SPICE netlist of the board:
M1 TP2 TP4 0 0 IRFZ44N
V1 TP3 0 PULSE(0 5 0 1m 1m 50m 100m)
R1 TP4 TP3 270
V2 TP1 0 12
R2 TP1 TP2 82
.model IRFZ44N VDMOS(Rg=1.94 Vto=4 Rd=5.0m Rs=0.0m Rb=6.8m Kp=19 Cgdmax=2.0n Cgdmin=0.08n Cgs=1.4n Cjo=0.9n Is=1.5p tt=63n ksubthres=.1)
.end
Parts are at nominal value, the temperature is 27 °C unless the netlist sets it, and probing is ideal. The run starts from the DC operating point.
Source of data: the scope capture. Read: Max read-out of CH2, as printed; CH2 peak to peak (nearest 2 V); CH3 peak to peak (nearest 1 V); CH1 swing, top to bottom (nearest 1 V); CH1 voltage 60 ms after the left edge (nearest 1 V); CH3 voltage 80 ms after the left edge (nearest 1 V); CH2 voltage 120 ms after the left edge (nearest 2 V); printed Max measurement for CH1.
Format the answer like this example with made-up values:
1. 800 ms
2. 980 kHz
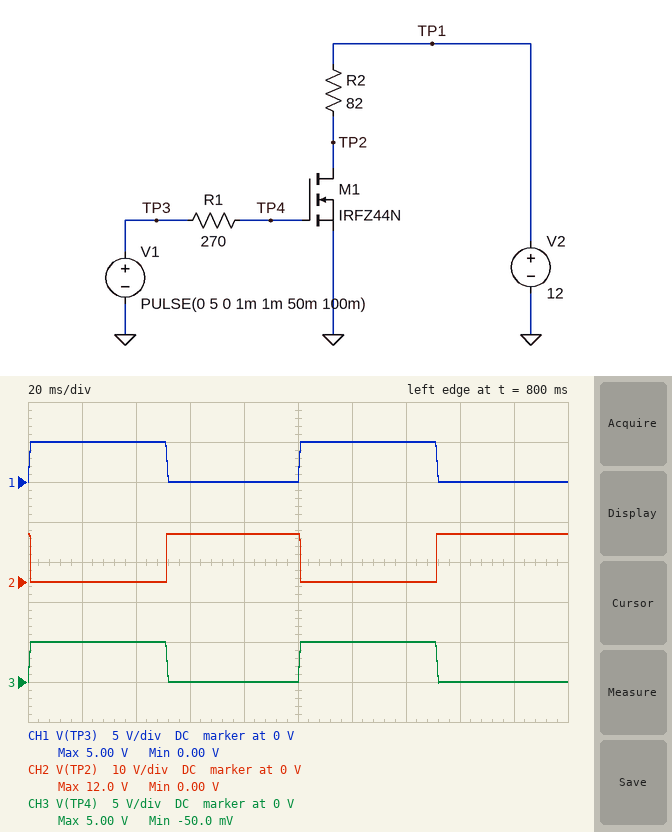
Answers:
1. 12.0 V
2. 12 V
3. 5 V
4. 5 V
5. 0 V
6. 0 V
7. 0 V
8. 5.00 V
